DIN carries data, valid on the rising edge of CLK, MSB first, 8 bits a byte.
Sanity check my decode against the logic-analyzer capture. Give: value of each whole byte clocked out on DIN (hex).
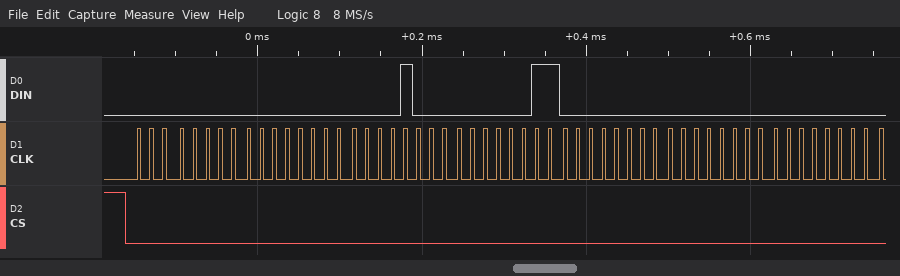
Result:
0x00 0x00 0x08 0x03 0x00 0x00 0x00
